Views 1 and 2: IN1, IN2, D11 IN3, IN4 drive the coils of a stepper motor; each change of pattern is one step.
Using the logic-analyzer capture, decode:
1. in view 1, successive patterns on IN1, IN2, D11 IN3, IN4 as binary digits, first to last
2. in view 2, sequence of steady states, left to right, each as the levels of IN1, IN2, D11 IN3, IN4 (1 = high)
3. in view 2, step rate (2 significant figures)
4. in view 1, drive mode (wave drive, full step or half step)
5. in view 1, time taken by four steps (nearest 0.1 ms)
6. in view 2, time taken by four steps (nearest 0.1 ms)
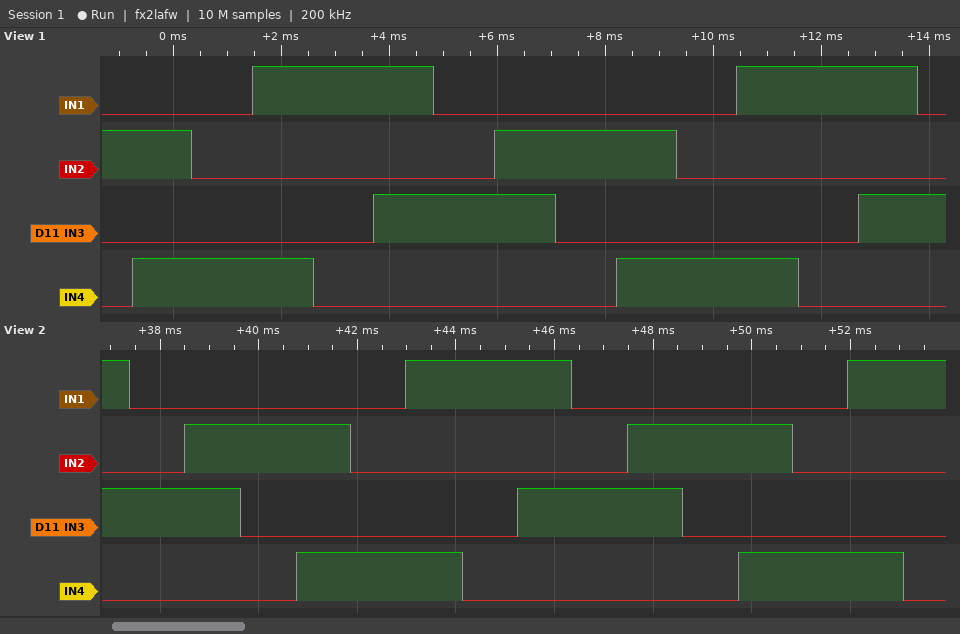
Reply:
0100 0101 0001 1001 1000 1010 0010 0110 0100 0101 0001 1001 1000 1010 0010
1010 0010 0110 0100 0101 0001 1001 1000 1010 0010 0110 0100 0101 0001 1001 1000
890 steps/s
half step
4.5 ms
4.5 ms
